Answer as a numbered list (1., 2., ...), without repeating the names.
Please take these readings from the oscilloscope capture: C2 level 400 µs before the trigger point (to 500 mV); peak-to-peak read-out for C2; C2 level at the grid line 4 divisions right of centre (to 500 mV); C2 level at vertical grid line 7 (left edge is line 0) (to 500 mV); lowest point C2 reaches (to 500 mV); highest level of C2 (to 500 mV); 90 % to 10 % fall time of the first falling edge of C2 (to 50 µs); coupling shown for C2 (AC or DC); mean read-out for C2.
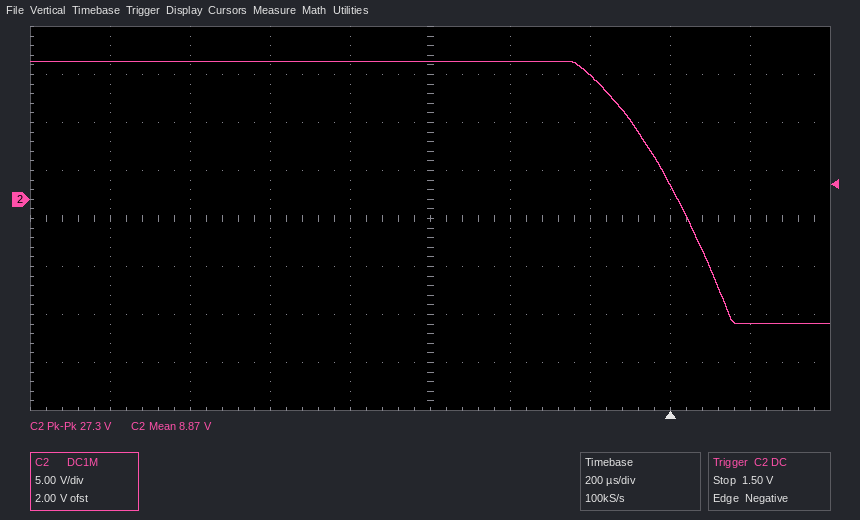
1. 14.5 V
2. 27.3 V
3. -13.0 V
4. 13.0 V
5. -13.0 V
6. 14.5 V
7. 300 µs
8. DC
9. 8.87 V
